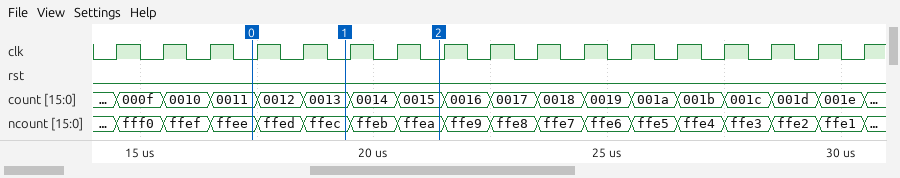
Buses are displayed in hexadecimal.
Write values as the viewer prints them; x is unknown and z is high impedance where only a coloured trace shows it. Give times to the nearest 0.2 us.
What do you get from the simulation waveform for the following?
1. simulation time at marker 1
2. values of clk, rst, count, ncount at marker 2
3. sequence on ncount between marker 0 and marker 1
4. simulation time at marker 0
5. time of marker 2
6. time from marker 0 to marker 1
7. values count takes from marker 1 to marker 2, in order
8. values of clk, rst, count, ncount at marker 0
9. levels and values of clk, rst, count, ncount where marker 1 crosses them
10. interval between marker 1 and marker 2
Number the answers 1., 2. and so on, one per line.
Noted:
1. 19.4 us
2. clk=0, rst=0, count=0015, ncount=ffea
3. ffee, ffed, ffec
4. 17.4 us
5. 21.4 us
6. 2 us
7. 0013, 0014, 0015
8. clk=0, rst=0, count=0011, ncount=ffee
9. clk=0, rst=0, count=0013, ncount=ffec
10. 2 us
